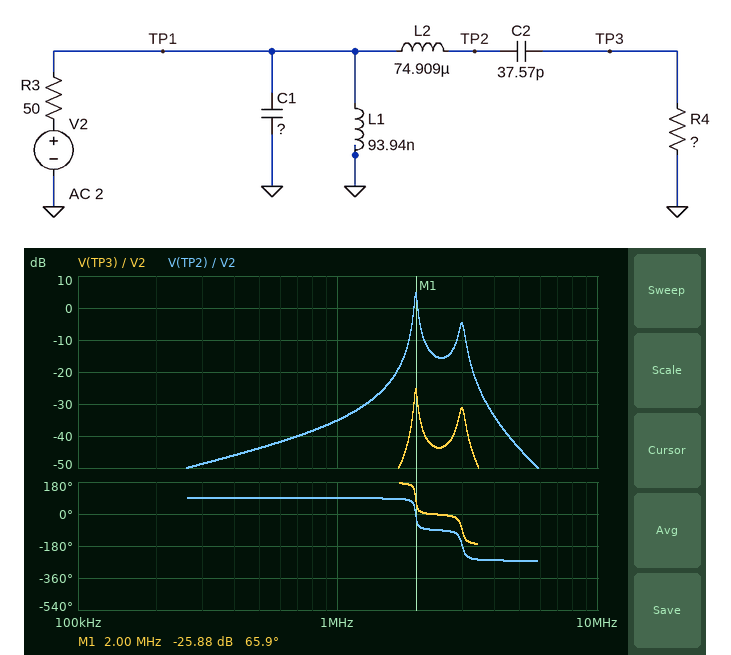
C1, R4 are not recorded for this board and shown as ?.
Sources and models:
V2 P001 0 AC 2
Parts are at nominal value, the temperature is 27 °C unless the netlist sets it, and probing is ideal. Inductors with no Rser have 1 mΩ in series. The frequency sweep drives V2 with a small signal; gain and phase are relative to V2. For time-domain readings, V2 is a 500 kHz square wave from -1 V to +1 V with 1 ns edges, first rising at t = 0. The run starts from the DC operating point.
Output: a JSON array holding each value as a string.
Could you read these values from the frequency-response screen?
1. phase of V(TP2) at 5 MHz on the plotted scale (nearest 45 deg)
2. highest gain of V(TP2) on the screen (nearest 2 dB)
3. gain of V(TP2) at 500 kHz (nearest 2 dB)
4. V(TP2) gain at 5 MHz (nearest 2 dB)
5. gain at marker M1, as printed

["-270 deg", "4 dB", "-44 dB", "-44 dB", "-25.88 dB"]
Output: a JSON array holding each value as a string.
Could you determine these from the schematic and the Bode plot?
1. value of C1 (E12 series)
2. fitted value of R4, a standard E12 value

["68 nF", "68 Ω"]
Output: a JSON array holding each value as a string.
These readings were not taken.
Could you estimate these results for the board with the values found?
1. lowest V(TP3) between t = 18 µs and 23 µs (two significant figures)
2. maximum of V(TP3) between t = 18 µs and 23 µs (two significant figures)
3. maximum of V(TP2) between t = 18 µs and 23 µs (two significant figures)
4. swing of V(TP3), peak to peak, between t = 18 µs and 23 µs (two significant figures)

["-2.6 mV", "2.7 mV", "67 mV", "5.3 mV"]
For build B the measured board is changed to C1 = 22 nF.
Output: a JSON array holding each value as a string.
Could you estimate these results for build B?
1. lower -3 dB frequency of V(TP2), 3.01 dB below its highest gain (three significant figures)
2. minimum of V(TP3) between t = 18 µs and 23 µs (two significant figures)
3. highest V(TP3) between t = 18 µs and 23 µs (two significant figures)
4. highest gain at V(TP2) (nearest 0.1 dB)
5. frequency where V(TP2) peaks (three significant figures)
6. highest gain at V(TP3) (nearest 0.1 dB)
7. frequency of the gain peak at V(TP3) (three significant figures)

["2.94 MHz", "-28 mV", "28 mV", "8.6 dB", "3.00 MHz", "-16.6 dB", "3.50 MHz"]
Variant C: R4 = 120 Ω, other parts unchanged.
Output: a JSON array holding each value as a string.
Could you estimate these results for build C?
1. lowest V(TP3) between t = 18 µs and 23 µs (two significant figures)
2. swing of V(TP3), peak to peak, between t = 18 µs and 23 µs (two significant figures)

["-4.5 mV", "9.1 mV"]
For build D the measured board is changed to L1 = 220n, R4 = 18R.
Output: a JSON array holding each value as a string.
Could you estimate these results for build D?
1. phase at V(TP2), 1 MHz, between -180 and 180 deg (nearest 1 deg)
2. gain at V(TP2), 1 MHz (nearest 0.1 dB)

["86 deg", "-22.4 dB"]
